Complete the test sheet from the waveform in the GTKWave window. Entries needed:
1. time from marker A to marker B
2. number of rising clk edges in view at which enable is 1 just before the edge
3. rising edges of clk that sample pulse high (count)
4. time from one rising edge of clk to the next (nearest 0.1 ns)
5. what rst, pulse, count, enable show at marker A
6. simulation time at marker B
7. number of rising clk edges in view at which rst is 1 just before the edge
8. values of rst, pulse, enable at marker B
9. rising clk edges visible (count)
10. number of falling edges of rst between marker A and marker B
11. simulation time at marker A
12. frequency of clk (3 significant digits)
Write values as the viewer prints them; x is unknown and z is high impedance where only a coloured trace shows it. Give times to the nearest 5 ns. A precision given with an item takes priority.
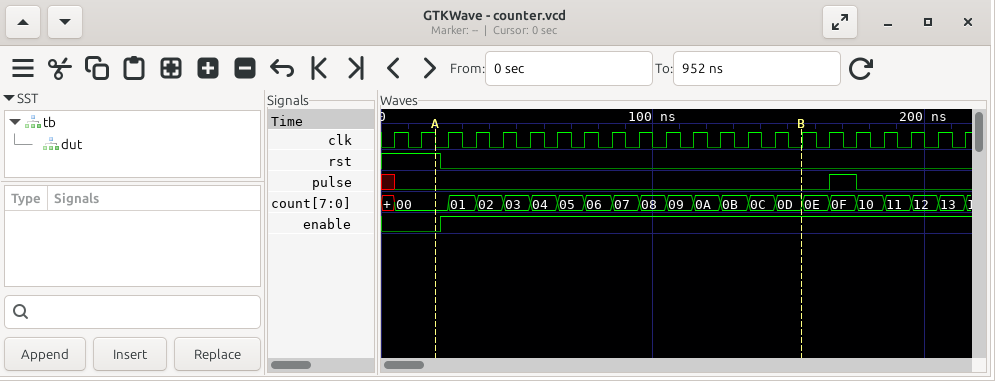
135 ns
20
1
10 ns
rst=1, pulse=0, count=00, enable=0
155 ns
2
rst=0, pulse=0, enable=1
22
1
20 ns
100 MHz
